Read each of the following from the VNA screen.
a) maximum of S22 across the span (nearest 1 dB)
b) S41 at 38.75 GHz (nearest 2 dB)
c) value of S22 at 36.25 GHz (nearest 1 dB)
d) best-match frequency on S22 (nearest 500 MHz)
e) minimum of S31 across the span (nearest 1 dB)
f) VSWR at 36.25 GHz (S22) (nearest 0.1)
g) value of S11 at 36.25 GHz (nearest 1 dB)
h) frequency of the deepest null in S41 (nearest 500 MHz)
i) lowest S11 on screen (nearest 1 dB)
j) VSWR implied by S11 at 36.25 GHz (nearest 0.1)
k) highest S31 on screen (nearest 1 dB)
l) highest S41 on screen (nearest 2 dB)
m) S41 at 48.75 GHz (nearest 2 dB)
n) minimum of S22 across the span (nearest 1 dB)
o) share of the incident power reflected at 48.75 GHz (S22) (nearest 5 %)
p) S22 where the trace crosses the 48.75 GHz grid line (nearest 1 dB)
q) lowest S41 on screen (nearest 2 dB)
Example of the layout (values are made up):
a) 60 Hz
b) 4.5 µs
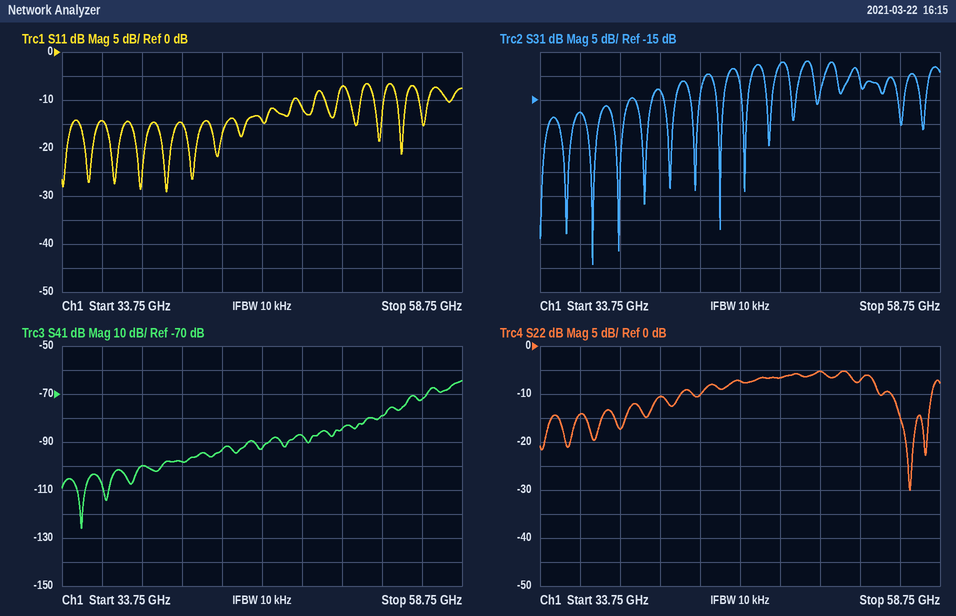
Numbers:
a) -5 dB
b) -100 dB
c) -14 dB
d) 57.0 GHz
e) -49 dB
f) 1.5
g) -14 dB
h) 35.0 GHz
i) -29 dB
j) 1.5
k) -7 dB
l) -64 dB
m) -88 dB
n) -30 dB
o) 20 %
p) -7 dB
q) -126 dB
